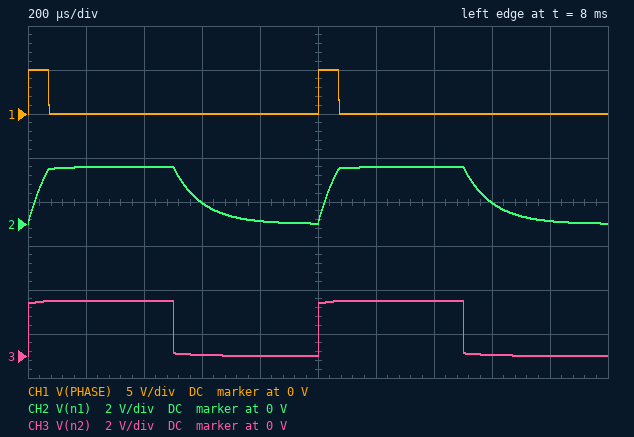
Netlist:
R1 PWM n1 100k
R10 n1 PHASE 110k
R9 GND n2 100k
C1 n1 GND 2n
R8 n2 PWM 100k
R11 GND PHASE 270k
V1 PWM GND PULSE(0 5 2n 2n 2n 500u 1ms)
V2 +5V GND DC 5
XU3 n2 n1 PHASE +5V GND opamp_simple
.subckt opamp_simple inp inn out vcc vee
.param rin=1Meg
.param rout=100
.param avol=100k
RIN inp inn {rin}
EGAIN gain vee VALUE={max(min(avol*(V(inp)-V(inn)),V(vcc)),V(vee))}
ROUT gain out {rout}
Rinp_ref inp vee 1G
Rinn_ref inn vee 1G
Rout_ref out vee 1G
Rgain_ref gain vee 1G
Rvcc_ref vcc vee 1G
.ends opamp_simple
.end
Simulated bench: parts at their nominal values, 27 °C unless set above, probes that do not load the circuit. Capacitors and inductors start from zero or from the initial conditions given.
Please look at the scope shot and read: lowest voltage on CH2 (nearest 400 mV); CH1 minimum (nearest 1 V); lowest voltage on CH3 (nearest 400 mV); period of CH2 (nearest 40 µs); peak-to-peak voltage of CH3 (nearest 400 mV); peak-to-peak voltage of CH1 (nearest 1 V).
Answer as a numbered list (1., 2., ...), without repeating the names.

1. 0 V
2. 0 V
3. 0 V
4. 1.00 ms
5. 2.4 V
6. 5 V
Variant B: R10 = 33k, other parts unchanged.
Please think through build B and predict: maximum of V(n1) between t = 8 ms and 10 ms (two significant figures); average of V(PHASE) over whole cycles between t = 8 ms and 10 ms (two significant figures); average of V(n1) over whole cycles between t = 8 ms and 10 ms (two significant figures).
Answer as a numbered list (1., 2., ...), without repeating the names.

1. 2.5 V
2. 950 mV
3. 1.3 V
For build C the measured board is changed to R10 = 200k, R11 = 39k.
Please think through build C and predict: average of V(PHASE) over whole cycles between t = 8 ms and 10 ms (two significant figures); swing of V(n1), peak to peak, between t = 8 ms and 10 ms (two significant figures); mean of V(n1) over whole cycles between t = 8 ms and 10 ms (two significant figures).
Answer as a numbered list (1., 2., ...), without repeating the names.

1. 450 mV
2. 3.2 V
3. 1.8 V
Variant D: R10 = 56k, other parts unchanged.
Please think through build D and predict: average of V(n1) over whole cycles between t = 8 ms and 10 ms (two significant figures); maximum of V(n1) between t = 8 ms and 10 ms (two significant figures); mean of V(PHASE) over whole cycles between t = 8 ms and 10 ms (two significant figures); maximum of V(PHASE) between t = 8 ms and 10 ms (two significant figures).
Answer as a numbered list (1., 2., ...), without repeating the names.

1. 1.4 V
2. 2.5 V
3. 740 mV
4. 5.0 V
